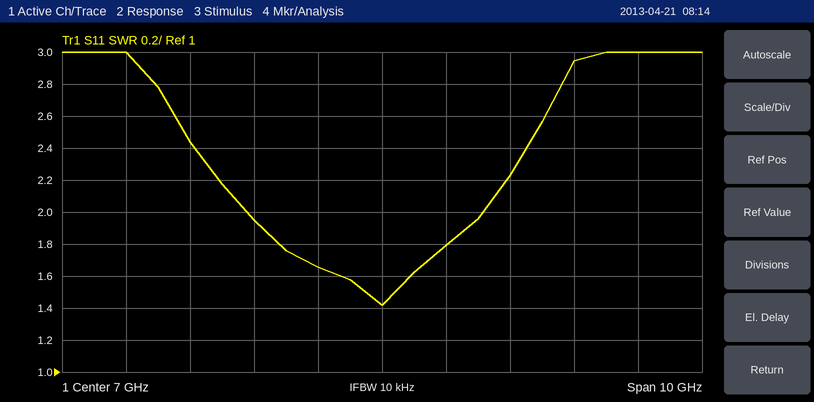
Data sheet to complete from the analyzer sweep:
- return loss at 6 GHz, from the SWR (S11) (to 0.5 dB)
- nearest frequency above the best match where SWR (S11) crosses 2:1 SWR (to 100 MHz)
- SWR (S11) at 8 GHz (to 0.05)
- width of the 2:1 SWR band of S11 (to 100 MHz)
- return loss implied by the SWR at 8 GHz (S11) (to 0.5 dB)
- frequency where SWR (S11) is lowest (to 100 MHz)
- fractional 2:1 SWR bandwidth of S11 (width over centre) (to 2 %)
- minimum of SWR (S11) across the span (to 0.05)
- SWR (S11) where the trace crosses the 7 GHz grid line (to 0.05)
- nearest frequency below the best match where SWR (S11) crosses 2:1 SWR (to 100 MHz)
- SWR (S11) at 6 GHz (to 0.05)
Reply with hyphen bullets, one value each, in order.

- 12.0 dB
- 8.6 GHz
- 1.80
- 3.7 GHz
- 11.0 dB
- 7.0 GHz
- 54 %
- 1.40
- 1.40
- 4.9 GHz
- 1.65
